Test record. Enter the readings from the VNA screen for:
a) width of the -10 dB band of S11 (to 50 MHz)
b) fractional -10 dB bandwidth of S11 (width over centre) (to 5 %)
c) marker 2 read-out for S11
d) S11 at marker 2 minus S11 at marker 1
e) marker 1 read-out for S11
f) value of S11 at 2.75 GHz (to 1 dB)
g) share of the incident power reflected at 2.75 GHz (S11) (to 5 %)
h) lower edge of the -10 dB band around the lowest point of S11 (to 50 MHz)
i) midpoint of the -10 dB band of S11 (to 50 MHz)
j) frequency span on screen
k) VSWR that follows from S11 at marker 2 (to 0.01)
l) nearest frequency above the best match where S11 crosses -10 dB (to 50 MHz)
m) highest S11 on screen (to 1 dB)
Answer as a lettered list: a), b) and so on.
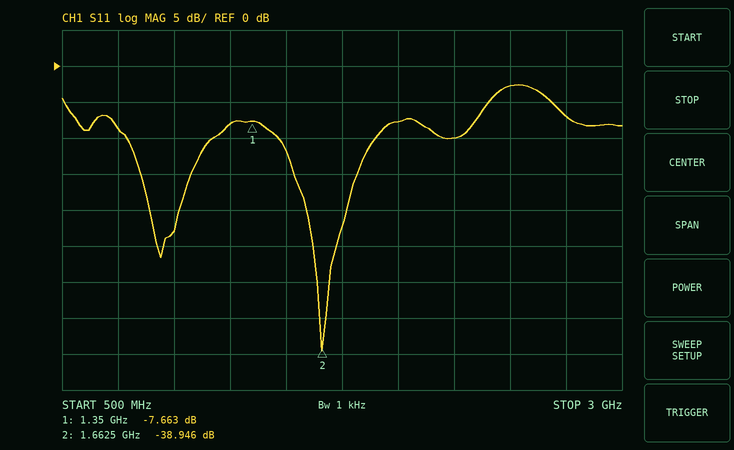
a) 450 MHz
b) 25 %
c) -38.946 dB
d) -31.283 dB
e) -7.663 dB
f) -7 dB
g) 20 %
h) 1.45 GHz
i) 1.70 GHz
j) 2.5 GHz
k) 1.02
l) 1.90 GHz
m) -3 dB
